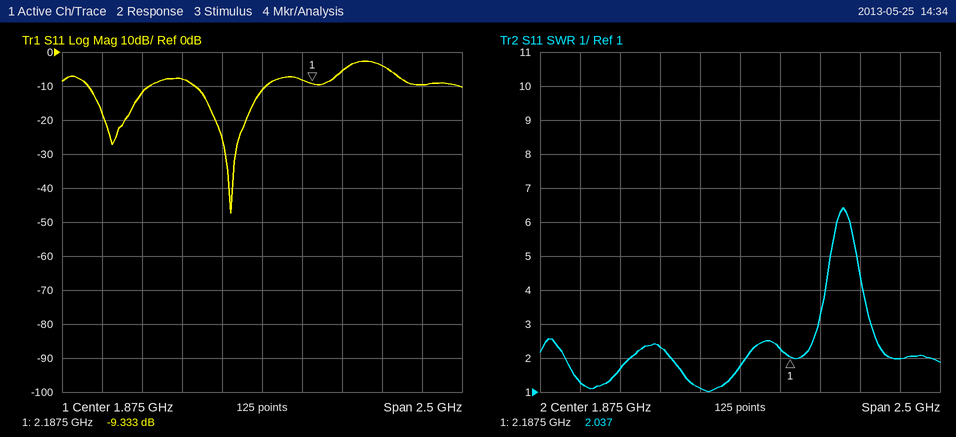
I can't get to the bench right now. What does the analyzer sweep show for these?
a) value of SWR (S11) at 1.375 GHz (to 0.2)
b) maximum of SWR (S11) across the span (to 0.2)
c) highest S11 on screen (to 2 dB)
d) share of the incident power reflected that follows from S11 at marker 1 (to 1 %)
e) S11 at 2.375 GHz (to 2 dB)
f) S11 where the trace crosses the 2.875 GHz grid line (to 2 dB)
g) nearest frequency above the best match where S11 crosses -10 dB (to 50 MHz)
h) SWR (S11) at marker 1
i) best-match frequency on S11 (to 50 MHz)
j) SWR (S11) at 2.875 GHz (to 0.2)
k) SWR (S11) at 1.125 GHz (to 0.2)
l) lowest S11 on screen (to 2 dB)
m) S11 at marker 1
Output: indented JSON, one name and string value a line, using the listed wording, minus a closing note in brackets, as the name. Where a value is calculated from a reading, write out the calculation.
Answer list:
{
  "value of SWR (S11) at 1.375 GHz": "2.4",
  "maximum of SWR (S11) across the span": "6.4",
  "highest S11 on screen": "-2 dB",
  "share of the incident power reflected that follows from S11 at marker 1": "10^(-9.333/10) ≈ 12 %",
  "S11 at 2.375 GHz": "-6 dB",
  "S11 where the trace crosses the 2.875 GHz grid line": "-10 dB",
  "nearest frequency above the best match where S11 crosses -10 dB": "1.90 GHz",
  "SWR (S11) at marker 1": "2.037",
  "best-match frequency on S11": "1.70 GHz",
  "SWR (S11) at 2.875 GHz": "2.0",
  "SWR (S11) at 1.125 GHz": "1.6",
  "lowest S11 on screen": "-48 dB",
  "S11 at marker 1": "-9.333 dB"
}
